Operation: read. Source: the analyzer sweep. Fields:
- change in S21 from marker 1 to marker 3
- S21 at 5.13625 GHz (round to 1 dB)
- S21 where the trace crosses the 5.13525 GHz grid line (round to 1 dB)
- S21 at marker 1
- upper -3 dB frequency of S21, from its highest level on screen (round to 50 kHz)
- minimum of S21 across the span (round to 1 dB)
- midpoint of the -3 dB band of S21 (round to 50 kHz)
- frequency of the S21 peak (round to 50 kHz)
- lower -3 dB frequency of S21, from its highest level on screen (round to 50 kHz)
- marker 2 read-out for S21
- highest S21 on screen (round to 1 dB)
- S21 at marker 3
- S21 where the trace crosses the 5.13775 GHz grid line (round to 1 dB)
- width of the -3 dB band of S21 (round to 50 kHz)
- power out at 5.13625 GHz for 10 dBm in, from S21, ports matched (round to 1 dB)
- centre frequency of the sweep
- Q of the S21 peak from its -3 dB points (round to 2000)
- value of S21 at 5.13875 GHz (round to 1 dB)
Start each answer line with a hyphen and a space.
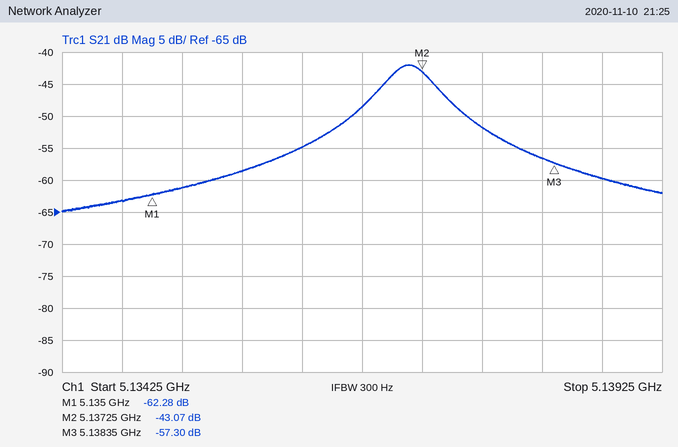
- 4.98 dB
- -55 dB
- -61 dB
- -62.28 dB
- 5.13735 GHz
- -65 dB
- 5.13715 GHz
- 5.13715 GHz
- 5.13695 GHz
- -43.07 dB
- -42 dB
- -57.30 dB
- -52 dB
- 400 kHz
- -45 dBm
- 5.13675 GHz
- 12000
- -60 dB
